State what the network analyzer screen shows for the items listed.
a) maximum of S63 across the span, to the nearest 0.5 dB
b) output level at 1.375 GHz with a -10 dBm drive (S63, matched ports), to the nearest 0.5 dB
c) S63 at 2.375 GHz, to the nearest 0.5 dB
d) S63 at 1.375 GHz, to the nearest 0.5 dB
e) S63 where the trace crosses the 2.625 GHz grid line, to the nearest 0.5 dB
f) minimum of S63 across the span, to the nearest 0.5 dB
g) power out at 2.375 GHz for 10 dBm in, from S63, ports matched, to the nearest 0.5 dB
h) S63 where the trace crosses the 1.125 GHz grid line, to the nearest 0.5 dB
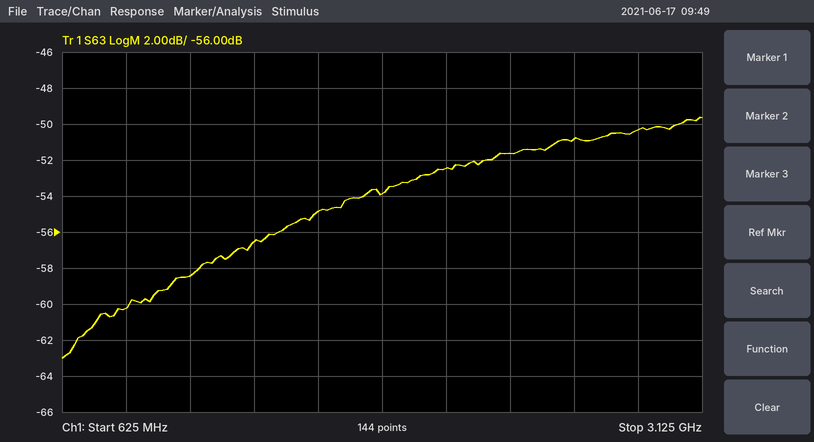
-49.5 dB
-66.5 dBm
-51.5 dB
-56.5 dB
-51.0 dB
-63.0 dB
-41.5 dBm
-58.5 dB
